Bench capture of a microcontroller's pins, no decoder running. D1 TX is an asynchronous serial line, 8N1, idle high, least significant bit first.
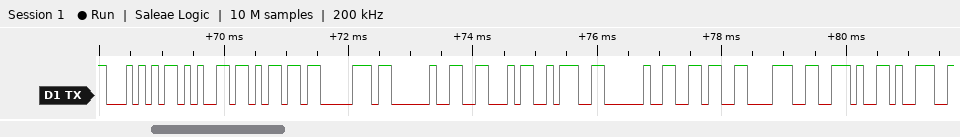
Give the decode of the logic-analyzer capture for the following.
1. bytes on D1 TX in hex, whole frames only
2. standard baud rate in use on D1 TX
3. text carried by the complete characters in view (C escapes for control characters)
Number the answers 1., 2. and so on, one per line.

1. 54 65 6D 70 20 46 3A 20 36 38 2E 39
2. 9600 baud
3. "Temp F: 68.9"
